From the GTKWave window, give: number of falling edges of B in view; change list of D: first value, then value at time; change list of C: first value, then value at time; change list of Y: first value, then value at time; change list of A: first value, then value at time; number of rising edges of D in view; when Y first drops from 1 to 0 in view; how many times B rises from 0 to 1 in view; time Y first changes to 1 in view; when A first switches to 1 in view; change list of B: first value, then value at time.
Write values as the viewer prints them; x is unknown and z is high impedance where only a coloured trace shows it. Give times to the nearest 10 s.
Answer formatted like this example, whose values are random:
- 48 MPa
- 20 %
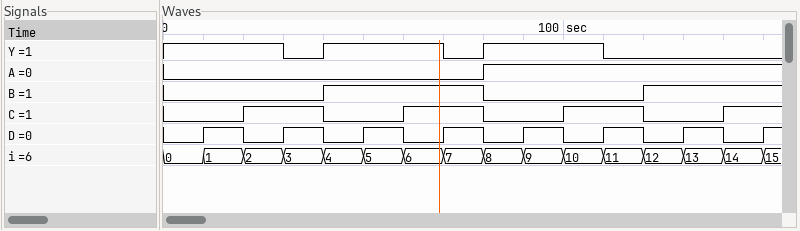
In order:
- 1
- 0, 1 at 10 s, 0 at 20 s, 1 at 30 s, 0 at 40 s, 1 at 50 s, 0 at 60 s, 1 at 70 s, 0 at 80 s, 1 at 90 s, 0 at 100 s, 1 at 110 s, 0 at 120 s, 1 at 130 s, 0 at 140 s, 1 at 150 s
- 0, 1 at 20 s, 0 at 40 s, 1 at 60 s, 0 at 80 s, 1 at 100 s, 0 at 120 s, 1 at 140 s
- 1, 0 at 30 s, 1 at 40 s, 0 at 70 s, 1 at 80 s, 0 at 110 s
- 0, 1 at 80 s
- 8
- 30 s
- 2
- 40 s
- 80 s
- 0, 1 at 40 s, 0 at 80 s, 1 at 120 s
